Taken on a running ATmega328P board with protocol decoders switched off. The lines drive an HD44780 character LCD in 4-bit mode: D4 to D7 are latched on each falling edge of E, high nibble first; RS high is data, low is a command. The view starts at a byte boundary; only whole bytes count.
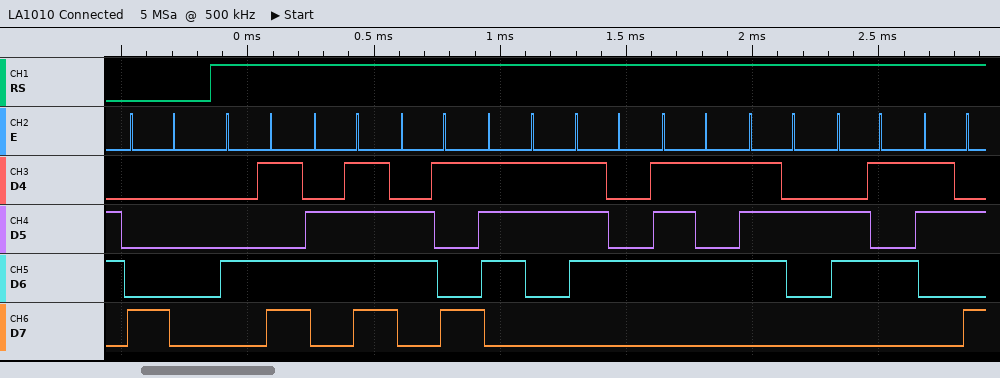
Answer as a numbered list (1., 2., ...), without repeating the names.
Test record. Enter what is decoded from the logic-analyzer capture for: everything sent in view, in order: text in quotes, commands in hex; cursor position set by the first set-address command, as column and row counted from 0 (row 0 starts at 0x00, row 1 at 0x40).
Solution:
1. 0x80 "Moisture:"
2. column 0, row 0
